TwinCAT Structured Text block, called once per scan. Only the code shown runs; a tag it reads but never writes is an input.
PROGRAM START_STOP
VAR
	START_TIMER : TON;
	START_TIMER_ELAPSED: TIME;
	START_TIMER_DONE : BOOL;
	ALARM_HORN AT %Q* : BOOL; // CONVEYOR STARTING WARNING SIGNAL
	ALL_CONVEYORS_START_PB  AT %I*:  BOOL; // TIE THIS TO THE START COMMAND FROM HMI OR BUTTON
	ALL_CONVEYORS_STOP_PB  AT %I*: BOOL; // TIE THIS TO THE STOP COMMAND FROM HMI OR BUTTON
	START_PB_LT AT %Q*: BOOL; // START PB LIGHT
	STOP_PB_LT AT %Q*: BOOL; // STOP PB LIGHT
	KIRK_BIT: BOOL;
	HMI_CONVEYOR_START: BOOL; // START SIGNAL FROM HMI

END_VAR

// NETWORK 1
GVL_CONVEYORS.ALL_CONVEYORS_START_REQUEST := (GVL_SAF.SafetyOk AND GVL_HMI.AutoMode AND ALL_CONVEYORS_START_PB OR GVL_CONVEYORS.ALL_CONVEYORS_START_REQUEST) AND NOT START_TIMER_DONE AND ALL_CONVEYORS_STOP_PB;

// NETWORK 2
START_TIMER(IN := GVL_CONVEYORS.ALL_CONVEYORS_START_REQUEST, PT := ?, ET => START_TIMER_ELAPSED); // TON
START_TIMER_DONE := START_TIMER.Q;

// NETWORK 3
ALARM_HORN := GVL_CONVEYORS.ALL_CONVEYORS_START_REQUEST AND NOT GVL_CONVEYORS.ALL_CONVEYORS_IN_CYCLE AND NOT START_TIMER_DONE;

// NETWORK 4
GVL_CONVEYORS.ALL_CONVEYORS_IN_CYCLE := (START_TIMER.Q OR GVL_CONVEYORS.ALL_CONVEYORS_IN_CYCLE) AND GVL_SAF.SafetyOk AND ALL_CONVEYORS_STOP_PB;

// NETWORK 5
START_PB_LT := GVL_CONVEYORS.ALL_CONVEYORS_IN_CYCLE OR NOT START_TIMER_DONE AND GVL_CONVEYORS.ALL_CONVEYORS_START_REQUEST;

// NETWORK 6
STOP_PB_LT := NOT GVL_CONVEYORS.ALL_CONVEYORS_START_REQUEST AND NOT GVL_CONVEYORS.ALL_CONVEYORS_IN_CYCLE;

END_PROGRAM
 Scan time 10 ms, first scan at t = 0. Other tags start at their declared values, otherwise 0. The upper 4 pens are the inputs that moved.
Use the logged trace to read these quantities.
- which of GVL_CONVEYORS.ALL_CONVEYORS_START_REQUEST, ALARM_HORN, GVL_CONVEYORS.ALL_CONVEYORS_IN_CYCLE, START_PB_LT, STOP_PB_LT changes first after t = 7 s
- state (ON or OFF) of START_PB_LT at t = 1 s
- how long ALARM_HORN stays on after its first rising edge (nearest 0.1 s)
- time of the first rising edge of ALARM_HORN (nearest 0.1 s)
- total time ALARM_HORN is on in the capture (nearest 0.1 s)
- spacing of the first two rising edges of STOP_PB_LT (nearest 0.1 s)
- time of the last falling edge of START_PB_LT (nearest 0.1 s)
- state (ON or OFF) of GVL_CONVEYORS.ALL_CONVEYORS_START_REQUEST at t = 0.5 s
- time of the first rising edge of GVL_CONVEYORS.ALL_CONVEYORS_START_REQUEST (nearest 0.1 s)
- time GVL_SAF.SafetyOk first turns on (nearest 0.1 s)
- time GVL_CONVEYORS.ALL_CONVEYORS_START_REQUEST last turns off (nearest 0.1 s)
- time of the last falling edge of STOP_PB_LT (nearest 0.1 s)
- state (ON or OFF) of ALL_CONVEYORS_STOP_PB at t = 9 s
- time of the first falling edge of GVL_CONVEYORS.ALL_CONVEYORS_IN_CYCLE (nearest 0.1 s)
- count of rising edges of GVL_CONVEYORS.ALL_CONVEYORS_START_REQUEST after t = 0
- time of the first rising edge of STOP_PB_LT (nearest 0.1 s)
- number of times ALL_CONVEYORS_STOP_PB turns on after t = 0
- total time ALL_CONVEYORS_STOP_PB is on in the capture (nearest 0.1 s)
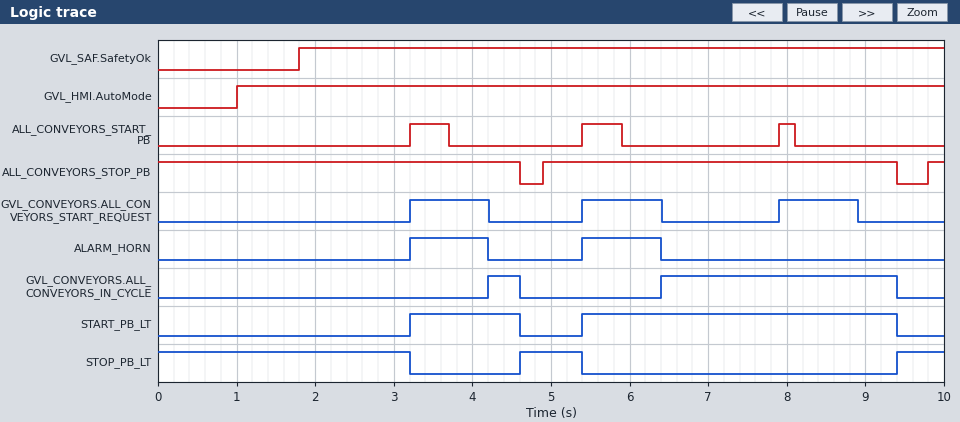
GVL_CONVEYORS.ALL_CONVEYORS_START_REQUEST
OFF
1.0 s
3.2 s
2.0 s
4.8 s
9.4 s
OFF
3.2 s
1.8 s
8.9 s
5.4 s
ON
4.6 s
3
4.6 s
2
9.3 s
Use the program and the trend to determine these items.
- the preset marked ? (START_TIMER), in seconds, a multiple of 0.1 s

1.0 s
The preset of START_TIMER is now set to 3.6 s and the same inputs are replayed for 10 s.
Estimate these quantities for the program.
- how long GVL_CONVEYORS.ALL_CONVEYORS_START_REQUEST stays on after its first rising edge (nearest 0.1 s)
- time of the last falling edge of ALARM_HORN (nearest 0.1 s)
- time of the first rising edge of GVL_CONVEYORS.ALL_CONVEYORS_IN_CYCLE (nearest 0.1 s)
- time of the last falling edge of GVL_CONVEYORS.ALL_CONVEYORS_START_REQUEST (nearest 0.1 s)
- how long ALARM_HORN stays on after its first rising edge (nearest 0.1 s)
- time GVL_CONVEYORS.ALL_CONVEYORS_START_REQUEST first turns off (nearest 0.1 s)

1.4 s
9.0 s
9.0 s
9.0 s
1.4 s
4.6 s
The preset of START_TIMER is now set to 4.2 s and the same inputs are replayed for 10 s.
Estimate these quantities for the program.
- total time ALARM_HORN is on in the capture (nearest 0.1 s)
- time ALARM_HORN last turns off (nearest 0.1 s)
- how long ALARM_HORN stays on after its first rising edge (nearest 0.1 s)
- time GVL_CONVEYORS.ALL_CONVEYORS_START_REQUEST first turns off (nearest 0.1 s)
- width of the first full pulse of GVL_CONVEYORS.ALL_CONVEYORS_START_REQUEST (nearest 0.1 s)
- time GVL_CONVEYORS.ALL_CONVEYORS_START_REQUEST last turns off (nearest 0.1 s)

5.4 s
9.4 s
1.4 s
4.6 s
1.4 s
9.4 s
